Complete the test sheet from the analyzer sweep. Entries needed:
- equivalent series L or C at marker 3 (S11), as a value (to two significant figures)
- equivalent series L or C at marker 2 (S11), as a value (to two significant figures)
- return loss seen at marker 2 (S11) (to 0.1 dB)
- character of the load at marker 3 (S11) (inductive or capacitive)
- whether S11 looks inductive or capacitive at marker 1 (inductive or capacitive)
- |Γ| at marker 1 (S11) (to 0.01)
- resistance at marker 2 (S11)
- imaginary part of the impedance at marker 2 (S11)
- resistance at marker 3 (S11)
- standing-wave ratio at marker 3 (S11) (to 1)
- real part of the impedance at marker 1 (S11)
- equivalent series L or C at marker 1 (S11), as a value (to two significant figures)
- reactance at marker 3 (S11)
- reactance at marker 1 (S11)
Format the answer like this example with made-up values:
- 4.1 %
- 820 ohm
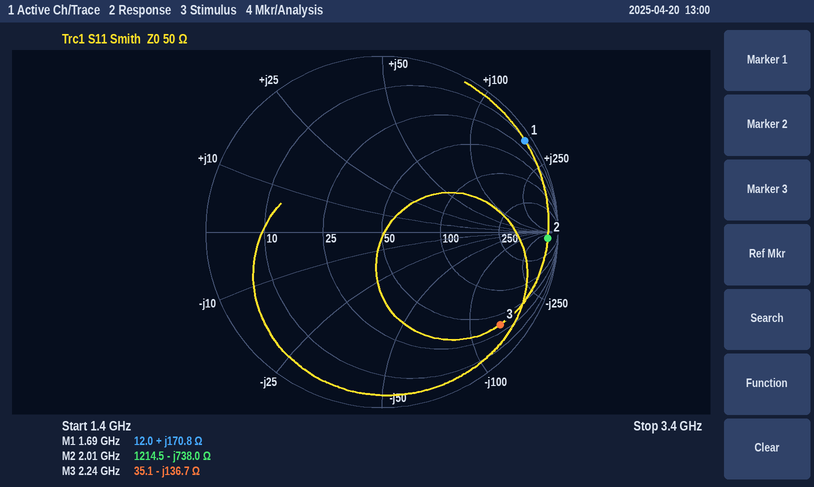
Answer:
- 520 fF
- 110 fF
- 0.5 dB
- capacitive
- inductive
- 0.96
- 1214.5 Ω
- -738.0 Ω
- 35.1 Ω
- 13
- 12.0 Ω
- 16 nH
- -136.7 Ω
- +170.8 Ω
